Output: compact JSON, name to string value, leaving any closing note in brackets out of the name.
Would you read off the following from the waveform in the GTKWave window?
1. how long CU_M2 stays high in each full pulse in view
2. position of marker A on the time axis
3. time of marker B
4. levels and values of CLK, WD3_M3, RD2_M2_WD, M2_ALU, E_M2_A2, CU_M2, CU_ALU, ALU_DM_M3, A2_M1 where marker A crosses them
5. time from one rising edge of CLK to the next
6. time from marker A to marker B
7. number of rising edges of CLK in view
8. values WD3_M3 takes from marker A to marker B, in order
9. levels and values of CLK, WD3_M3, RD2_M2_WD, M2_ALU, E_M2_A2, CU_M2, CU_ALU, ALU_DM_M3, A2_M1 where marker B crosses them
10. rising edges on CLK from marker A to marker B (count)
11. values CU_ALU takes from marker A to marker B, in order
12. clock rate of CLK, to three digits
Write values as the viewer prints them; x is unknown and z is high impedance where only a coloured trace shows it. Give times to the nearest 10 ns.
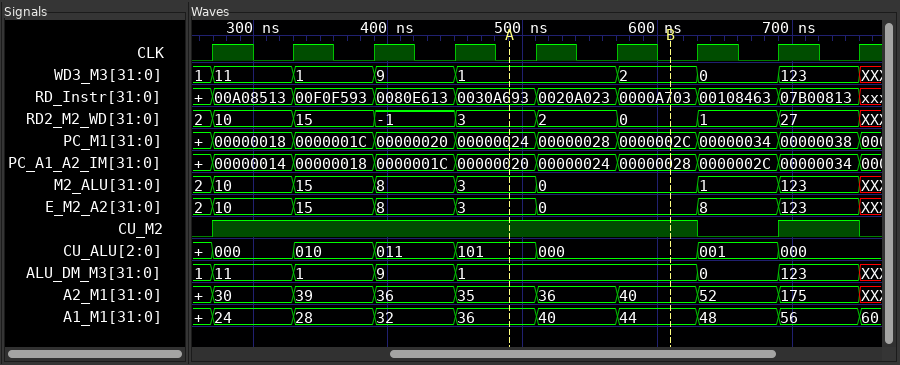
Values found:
{"how long CU_M2 stays high in each full pulse in view": "360 ns, 60 ns", "position of marker A on the time axis": "490 ns", "time of marker B": "610 ns", "levels and values of CLK, WD3_M3, RD2_M2_WD, M2_ALU, E_M2_A2, CU_M2, CU_ALU, ALU_DM_M3, A2_M1 where marker A crosses them": "CLK=0, WD3_M3=1, RD2_M2_WD=3, M2_ALU=3, E_M2_A2=3, CU_M2=1, CU_ALU=101, ALU_DM_M3=1, A2_M1=35", "time from one rising edge of CLK to the next": "60 ns", "time from marker A to marker B": "120 ns", "number of rising edges of CLK in view": "9", "values WD3_M3 takes from marker A to marker B, in order": "1, 2", "levels and values of CLK, WD3_M3, RD2_M2_WD, M2_ALU, E_M2_A2, CU_M2, CU_ALU, ALU_DM_M3, A2_M1 where marker B crosses them": "CLK=0, WD3_M3=2, RD2_M2_WD=0, M2_ALU=0, E_M2_A2=0, CU_M2=1, CU_ALU=000, ALU_DM_M3=1, A2_M1=40", "rising edges on CLK from marker A to marker B": "2", "values CU_ALU takes from marker A to marker B, in order": "101, 000", "clock rate of CLK, to three digits": "16.7 MHz"}
